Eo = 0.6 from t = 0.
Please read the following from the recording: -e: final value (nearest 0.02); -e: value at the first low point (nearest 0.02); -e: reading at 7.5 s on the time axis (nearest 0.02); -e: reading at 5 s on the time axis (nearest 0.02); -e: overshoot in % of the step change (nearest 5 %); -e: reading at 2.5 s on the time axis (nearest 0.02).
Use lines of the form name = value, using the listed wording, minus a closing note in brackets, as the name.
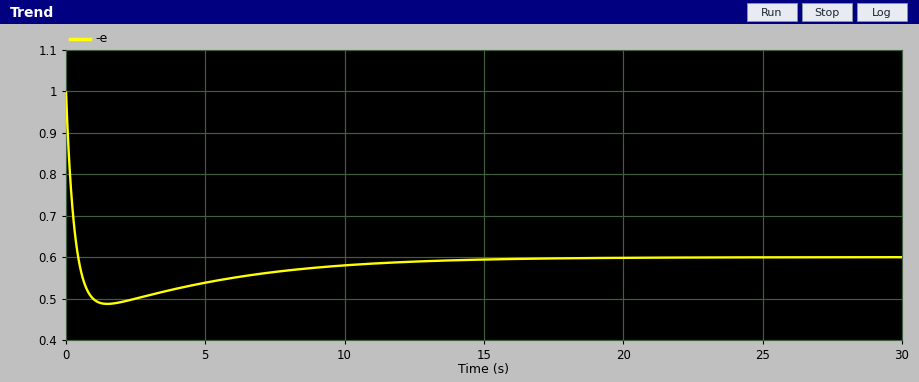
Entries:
-e: final value = 0.60
-e: value at the first low point = 0.48
-e: reading at 7.5 s on the time axis = 0.56
-e: reading at 5 s on the time axis = 0.54
-e: overshoot in % of the step change = 30 %
-e: reading at 2.5 s on the time axis = 0.50
